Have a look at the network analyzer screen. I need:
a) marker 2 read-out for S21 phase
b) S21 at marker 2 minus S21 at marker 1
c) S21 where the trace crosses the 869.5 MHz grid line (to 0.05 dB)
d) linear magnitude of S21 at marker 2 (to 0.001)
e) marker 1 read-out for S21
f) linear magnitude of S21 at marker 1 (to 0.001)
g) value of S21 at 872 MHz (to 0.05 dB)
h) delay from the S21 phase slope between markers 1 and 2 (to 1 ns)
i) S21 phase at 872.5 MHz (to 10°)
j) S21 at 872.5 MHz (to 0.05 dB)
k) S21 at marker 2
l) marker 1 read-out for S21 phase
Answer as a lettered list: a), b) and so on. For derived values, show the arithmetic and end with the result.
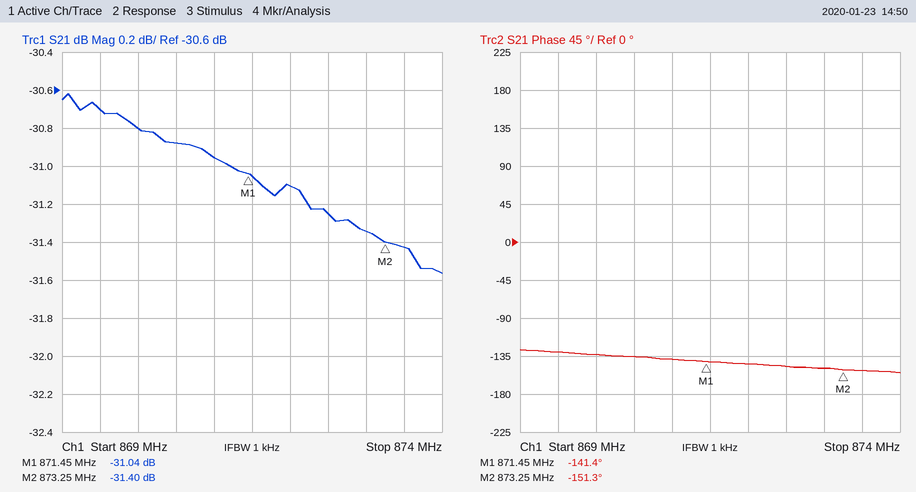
a) -151.3°
b) -31.4 − (-31.04) = -0.36 dB
c) -30.70 dB
d) 10^(-31.4/20) ≈ 0.027
e) -31.04 dB
f) 10^(-31.04/20) ≈ 0.028
g) -31.10 dB
h) −(-151.3° − (-141.4°))/(360° × 1.8 MHz) ≈ 15 ns
i) -150°
j) -31.25 dB
k) -31.40 dB
l) -141.4°
